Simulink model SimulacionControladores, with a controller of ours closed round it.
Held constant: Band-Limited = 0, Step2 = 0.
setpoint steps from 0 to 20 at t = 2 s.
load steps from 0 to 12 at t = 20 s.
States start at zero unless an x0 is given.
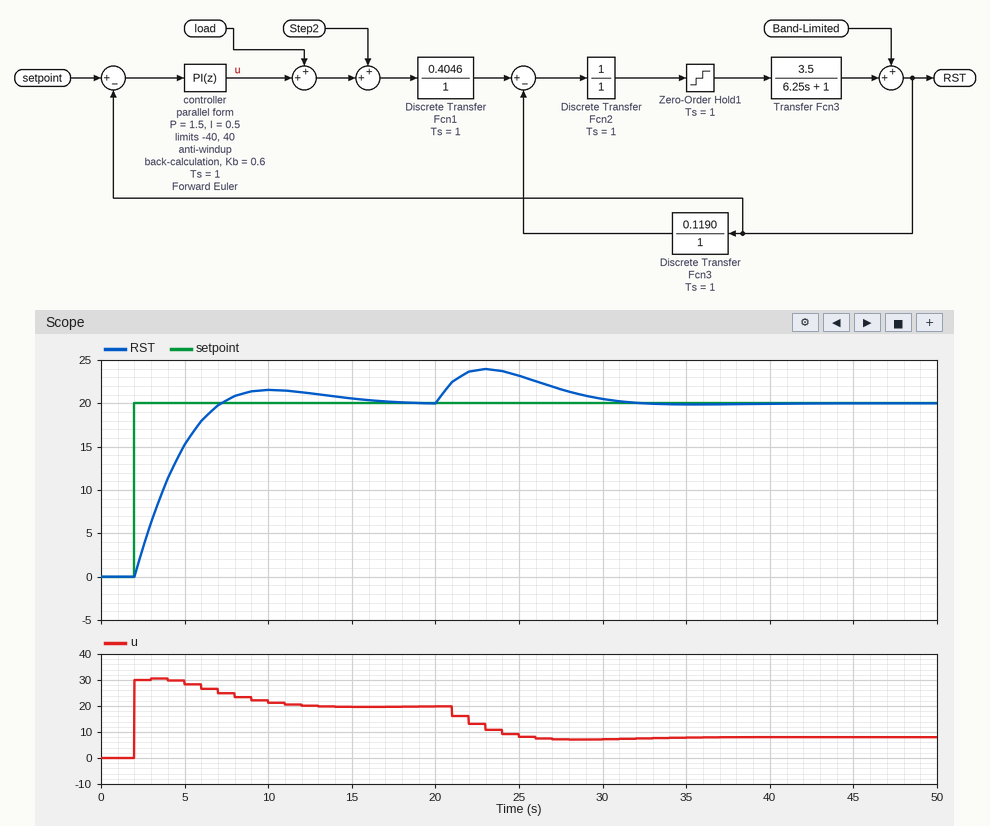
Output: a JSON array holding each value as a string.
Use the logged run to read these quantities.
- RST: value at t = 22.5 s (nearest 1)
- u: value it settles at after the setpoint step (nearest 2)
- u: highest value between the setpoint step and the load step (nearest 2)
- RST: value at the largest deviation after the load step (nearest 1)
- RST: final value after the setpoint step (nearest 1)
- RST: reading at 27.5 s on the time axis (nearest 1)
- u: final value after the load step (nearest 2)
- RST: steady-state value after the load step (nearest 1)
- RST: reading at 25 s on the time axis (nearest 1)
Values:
["24", "20", "30", "24", "20", "22", "8", "20", "23"]
